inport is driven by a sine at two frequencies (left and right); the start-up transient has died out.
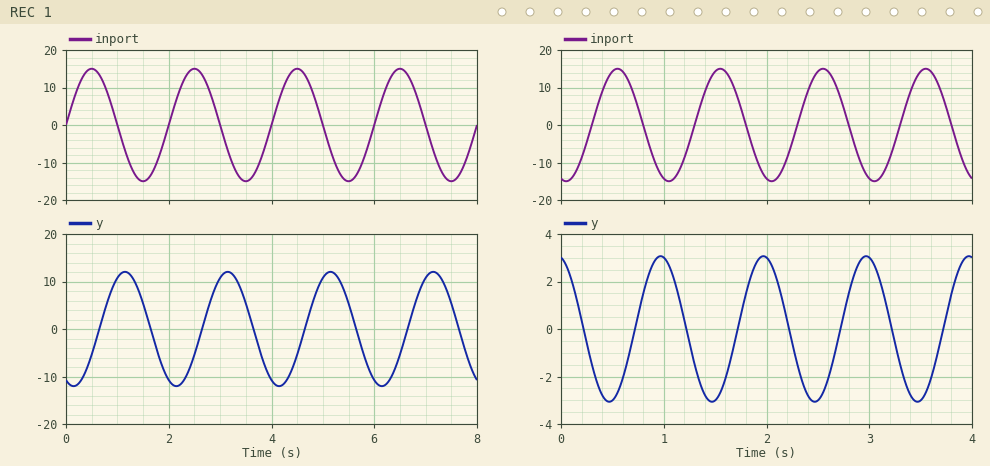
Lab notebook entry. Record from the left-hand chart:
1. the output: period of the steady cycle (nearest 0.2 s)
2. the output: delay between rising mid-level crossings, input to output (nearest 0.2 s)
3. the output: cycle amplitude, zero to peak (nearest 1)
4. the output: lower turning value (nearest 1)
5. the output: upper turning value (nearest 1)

2.0 s
0.6 s
12
-12
12
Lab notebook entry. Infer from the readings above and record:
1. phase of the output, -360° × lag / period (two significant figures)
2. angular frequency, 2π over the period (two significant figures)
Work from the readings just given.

-110°
3.1 rad/s
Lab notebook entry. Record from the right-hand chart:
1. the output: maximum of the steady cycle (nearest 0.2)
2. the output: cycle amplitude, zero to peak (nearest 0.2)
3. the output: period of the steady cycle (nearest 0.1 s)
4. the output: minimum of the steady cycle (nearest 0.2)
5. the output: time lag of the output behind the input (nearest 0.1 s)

3.0
3.0
1.0 s
-3.0
0.4 s
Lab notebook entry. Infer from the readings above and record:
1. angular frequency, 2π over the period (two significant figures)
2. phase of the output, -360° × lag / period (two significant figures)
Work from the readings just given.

6.3 rad/s
-140°
